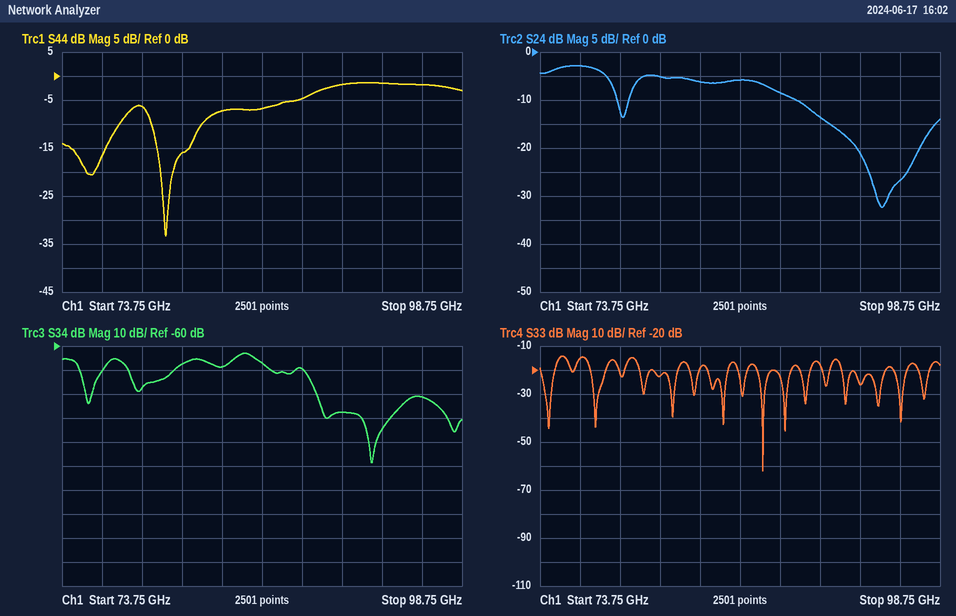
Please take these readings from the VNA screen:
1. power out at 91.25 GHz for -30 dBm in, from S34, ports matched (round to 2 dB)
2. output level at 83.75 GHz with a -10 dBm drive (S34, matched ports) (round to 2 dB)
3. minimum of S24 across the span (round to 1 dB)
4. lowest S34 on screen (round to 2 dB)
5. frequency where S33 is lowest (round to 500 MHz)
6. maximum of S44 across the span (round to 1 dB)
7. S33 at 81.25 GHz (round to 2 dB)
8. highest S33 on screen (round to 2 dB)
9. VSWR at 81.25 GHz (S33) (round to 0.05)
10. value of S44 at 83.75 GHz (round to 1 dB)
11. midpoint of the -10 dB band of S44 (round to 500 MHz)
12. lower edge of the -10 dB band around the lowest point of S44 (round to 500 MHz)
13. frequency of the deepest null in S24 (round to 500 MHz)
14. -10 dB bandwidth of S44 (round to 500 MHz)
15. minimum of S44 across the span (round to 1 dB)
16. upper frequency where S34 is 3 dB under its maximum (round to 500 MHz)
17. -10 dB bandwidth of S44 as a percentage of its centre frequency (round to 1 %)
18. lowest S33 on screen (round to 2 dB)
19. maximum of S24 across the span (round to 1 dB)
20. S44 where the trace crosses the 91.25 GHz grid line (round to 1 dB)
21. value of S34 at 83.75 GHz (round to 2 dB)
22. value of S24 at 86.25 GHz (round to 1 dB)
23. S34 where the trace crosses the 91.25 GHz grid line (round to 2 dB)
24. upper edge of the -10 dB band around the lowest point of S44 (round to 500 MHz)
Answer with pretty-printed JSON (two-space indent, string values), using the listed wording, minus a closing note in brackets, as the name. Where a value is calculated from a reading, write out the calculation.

{
  "power out at 91.25 GHz for -30 dBm in, from S34, ports matched": "-30 dBm + (-88 dB) = -118 dBm",
  "output level at 83.75 GHz with a -10 dBm drive (S34, matched ports)": "-10 dBm + (-68 dB) = -78 dBm",
  "minimum of S24 across the span": "-32 dB",
  "lowest S34 on screen": "-108 dB",
  "frequency where S33 is lowest": "87.5 GHz",
  "maximum of S44 across the span": "-1 dB",
  "S33 at 81.25 GHz": "-22 dB",
  "highest S33 on screen": "-14 dB",
  "VSWR at 81.25 GHz (S33)": "|Γ| = 10^(-22/20) = 0.0794; VSWR = (1 + 0.0794)/(1 − 0.0794) ≈ 1.17, so 1.15 to the nearest 0.05",
  "value of S44 at 83.75 GHz": "-7 dB",
  "midpoint of the -10 dB band of S44": "81.0 GHz",
  "lower edge of the -10 dB band around the lowest point of S44": "79.5 GHz",
  "frequency of the deepest null in S24": "95.0 GHz",
  "-10 dB bandwidth of S44": "82.5 GHz − 79.5 GHz = 3.0 GHz",
  "minimum of S44 across the span": "-33 dB",
  "upper frequency where S34 is 3 dB under its maximum": "86.0 GHz",
  "-10 dB bandwidth of S44 as a percentage of its centre frequency": "3 GHz / 81 GHz ≈ 4 %",
  "lowest S33 on screen": "-62 dB",
  "maximum of S24 across the span": "-3 dB",
  "S44 where the trace crosses the 91.25 GHz grid line": "-2 dB",
  "value of S34 at 83.75 GHz": "-68 dB",
  "value of S24 at 86.25 GHz": "-6 dB",
  "S34 where the trace crosses the 91.25 GHz grid line": "-88 dB",
  "upper edge of the -10 dB band around the lowest point of S44": "82.5 GHz"
}
